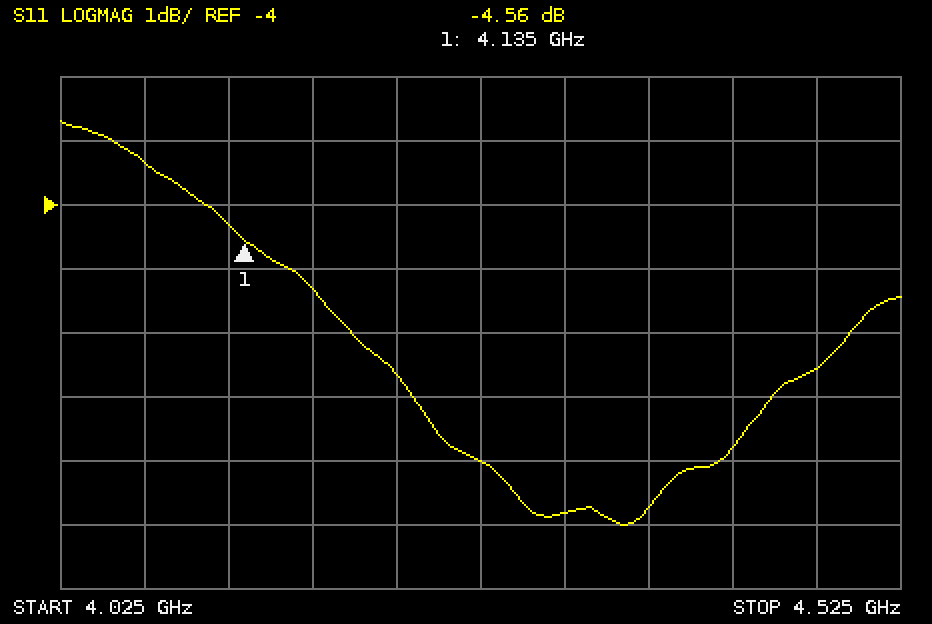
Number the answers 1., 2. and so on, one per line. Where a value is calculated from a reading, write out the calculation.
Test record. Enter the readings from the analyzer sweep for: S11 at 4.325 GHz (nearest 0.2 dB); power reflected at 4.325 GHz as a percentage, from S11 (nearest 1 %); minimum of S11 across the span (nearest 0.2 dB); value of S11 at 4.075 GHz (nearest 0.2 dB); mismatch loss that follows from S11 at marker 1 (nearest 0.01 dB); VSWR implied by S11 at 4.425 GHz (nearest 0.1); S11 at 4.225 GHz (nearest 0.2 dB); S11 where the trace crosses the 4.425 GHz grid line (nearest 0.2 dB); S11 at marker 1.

1. -8.8 dB
2. 10^(-8.8/10) ≈ 13 %
3. -9.0 dB
4. -3.4 dB
5. −10 log10(1 − 10^(-4.56/10)) ≈ 1.87 dB
6. |Γ| = 10^(-7.8/20) = 0.4074; VSWR = (1 + 0.4074)/(1 − 0.4074) ≈ 2.4
7. -6.6 dB
8. -7.8 dB
9. -4.56 dB
